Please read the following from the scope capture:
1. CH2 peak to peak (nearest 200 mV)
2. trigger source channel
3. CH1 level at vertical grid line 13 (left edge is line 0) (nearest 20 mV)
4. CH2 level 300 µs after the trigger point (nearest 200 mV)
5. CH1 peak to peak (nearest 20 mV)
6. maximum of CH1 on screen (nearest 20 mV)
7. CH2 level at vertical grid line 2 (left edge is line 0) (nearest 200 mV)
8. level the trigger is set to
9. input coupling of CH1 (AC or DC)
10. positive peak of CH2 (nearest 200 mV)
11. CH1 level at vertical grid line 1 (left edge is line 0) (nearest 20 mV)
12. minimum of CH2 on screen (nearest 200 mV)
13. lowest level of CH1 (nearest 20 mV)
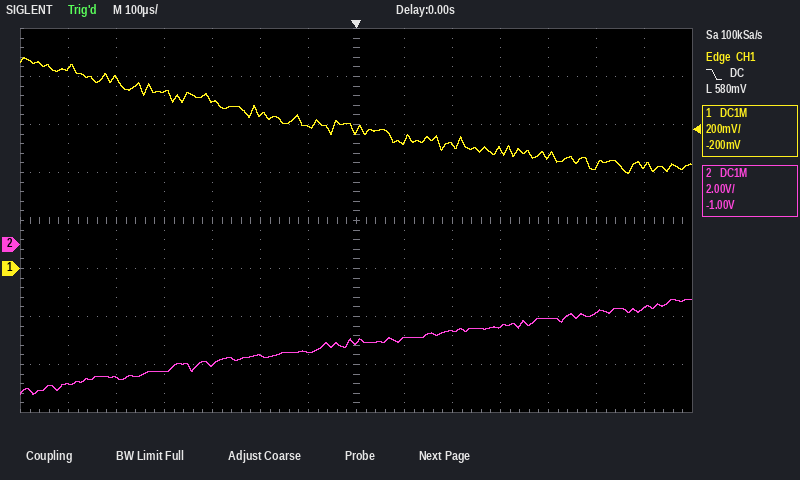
4.0 V
CH1
420 mV
-3.4 V
480 mV
880 mV
-5.6 V
580 mV
DC
-2.2 V
840 mV
-6.2 V
400 mV
